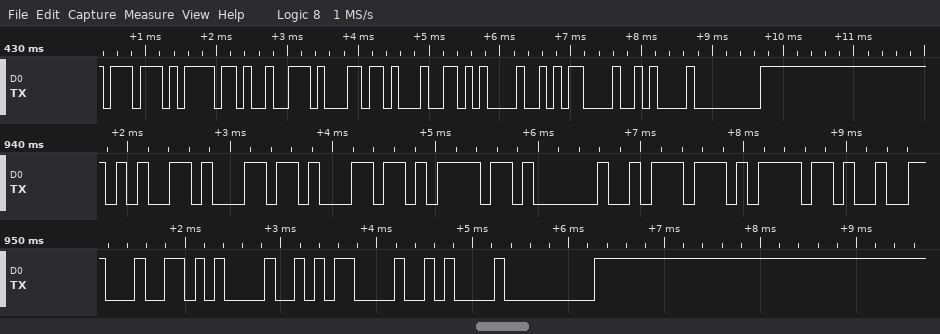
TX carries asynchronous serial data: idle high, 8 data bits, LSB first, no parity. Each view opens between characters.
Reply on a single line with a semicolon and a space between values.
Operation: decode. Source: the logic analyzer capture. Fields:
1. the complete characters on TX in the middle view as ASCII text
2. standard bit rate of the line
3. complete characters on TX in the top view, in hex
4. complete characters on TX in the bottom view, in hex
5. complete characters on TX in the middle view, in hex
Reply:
"ello wo"; 9600 baud; 77, 6F, 72, 6C, 64, 21, 0D, 0A, 00; 64, 21, 0D, 0A, 00; 65, 6C, 6C, 6F, 20, 77, 6F
